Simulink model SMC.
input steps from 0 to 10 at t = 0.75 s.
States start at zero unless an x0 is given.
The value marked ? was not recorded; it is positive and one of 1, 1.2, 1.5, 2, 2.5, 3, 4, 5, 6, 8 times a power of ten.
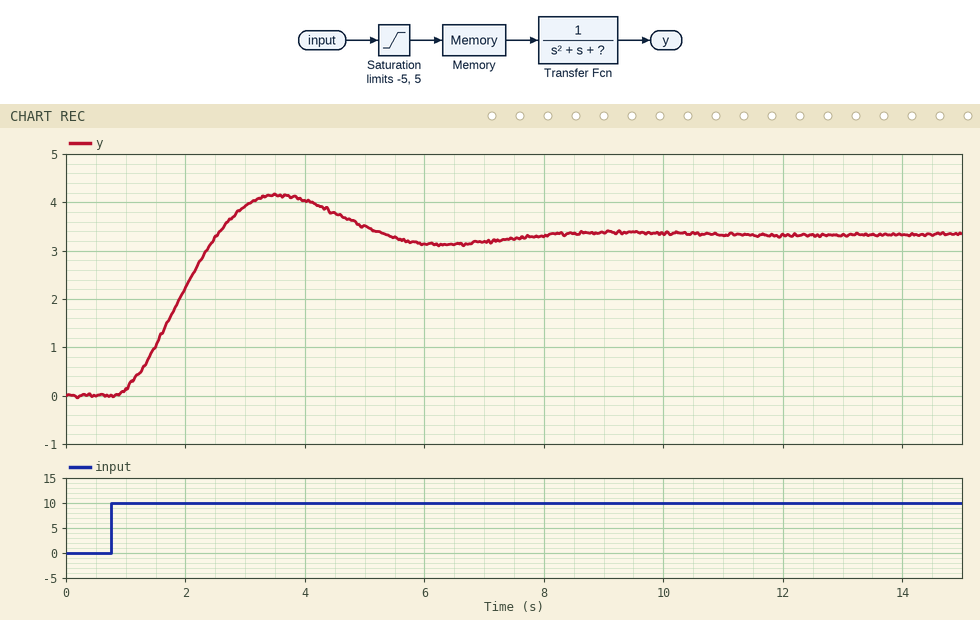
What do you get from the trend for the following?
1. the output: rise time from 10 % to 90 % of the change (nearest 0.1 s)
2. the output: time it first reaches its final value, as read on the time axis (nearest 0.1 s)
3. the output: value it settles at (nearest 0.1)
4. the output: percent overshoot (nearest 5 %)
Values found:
1.2 s
2.5 s
3.3
25 %
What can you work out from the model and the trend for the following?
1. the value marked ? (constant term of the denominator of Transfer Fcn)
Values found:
1.5
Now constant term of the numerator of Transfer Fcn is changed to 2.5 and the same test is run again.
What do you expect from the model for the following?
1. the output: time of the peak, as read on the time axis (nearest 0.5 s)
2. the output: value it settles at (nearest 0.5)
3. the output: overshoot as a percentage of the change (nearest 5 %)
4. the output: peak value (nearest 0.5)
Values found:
3.5 s
8.5
25 %
10.5
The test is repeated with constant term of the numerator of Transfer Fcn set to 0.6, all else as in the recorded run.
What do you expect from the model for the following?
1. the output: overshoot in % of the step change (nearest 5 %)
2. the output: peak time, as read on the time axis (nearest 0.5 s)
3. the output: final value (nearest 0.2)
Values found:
25 %
3.5 s
2.0
